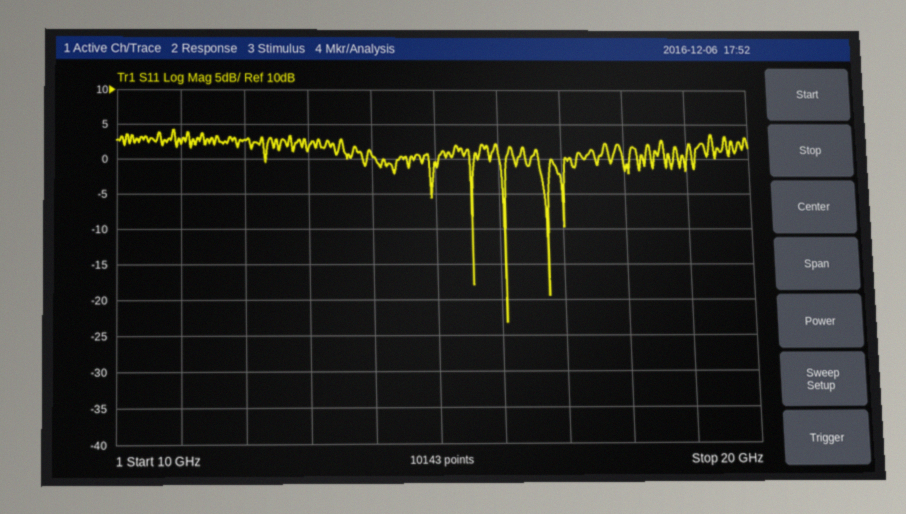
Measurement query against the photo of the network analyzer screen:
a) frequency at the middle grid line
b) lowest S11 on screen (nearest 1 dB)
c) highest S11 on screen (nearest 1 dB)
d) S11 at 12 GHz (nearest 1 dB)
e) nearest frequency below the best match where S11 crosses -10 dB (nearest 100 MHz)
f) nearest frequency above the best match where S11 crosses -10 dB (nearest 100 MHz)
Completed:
15 GHz
-23 dB
4 dB
3 dB
16.1 GHz
16.1 GHz
